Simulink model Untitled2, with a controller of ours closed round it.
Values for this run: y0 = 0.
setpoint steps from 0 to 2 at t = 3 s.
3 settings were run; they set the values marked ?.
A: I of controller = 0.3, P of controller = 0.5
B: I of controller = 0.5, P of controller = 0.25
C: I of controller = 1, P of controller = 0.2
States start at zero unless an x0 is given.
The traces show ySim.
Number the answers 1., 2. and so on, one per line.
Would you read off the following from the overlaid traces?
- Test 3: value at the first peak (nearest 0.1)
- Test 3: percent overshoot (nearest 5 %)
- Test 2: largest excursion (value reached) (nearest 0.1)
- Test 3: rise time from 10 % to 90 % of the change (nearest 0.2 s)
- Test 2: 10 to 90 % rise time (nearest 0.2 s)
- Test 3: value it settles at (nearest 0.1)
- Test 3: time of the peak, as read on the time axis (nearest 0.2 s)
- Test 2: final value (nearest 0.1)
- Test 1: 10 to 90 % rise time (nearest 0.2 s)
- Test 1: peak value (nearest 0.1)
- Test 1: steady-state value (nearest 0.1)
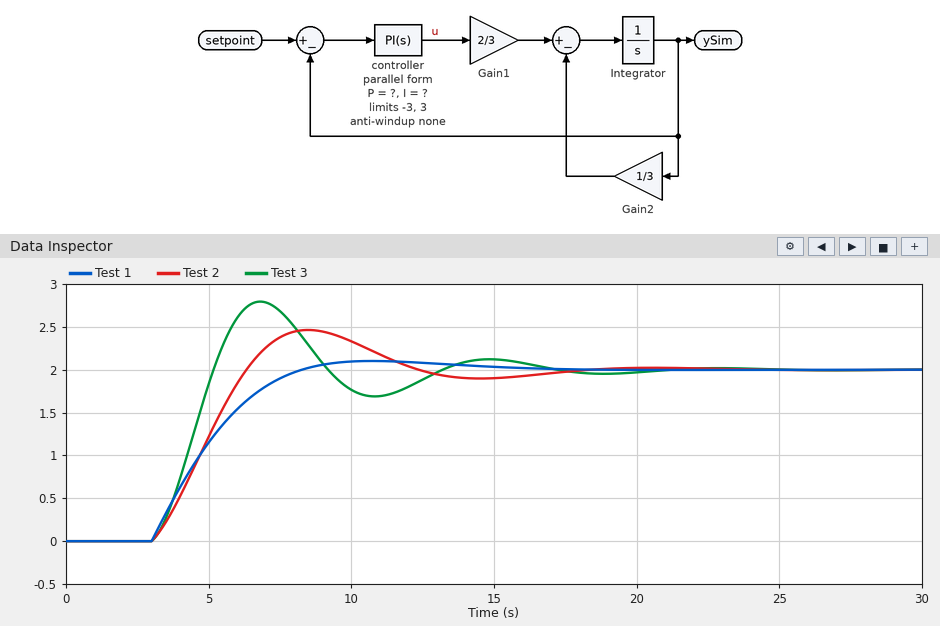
1. 2.8
2. 40 %
3. 2.5
4. 1.6 s
5. 2.4 s
6. 2.0
7. 6.8 s
8. 2.0
9. 3.6 s
10. 2.1
11. 2.0
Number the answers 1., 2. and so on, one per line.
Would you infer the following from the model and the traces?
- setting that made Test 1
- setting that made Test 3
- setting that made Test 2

1. A
2. C
3. B
